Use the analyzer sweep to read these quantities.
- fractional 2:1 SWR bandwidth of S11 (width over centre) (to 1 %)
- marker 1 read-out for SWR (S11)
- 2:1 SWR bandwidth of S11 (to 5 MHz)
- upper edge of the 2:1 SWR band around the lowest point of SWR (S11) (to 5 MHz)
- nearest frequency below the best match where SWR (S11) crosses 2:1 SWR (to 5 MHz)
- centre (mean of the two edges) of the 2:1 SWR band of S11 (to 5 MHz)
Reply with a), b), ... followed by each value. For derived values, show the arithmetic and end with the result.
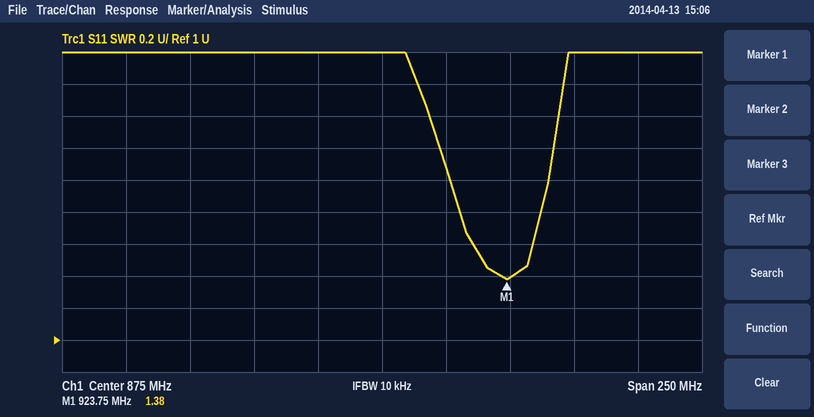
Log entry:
a) 40 MHz / 920 MHz ≈ 4 %
b) 1.38
c) 940 MHz − 900 MHz = 40 MHz
d) 940 MHz
e) 900 MHz
f) 920 MHz
